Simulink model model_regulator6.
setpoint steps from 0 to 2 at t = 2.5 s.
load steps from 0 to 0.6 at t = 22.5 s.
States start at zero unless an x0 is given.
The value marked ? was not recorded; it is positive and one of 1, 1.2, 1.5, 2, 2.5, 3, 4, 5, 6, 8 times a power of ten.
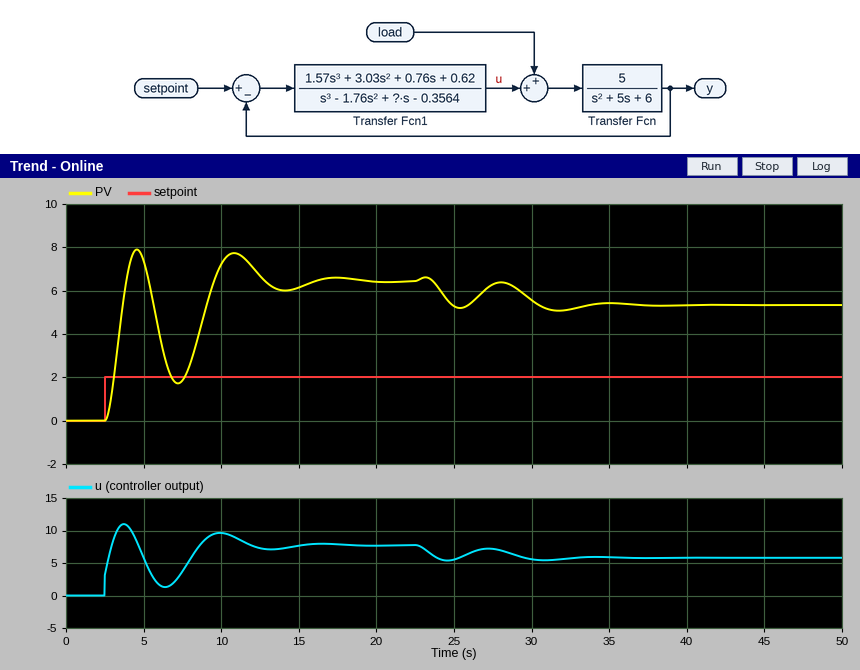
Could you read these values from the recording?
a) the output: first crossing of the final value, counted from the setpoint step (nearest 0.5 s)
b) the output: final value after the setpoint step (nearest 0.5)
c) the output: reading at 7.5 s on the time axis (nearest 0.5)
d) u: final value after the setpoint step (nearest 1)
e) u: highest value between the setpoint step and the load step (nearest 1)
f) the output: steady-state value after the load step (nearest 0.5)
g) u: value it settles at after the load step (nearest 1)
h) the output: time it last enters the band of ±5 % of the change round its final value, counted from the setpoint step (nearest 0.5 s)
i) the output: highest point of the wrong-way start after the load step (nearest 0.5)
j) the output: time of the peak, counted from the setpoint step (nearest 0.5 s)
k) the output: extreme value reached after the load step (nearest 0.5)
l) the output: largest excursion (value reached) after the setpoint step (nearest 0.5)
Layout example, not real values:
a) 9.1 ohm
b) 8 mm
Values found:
a) 1.5 s
b) 6.5
c) 2.0
d) 8
e) 11
f) 5.5
g) 6
h) 12.5 s
i) 6.5
j) 2.0 s
k) 5.0
l) 8.0
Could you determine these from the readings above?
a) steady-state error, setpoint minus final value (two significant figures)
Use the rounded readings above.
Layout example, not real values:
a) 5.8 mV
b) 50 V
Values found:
a) -4.5
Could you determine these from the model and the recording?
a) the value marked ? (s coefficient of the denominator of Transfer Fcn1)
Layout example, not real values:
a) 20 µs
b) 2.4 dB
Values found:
a) 0.2
